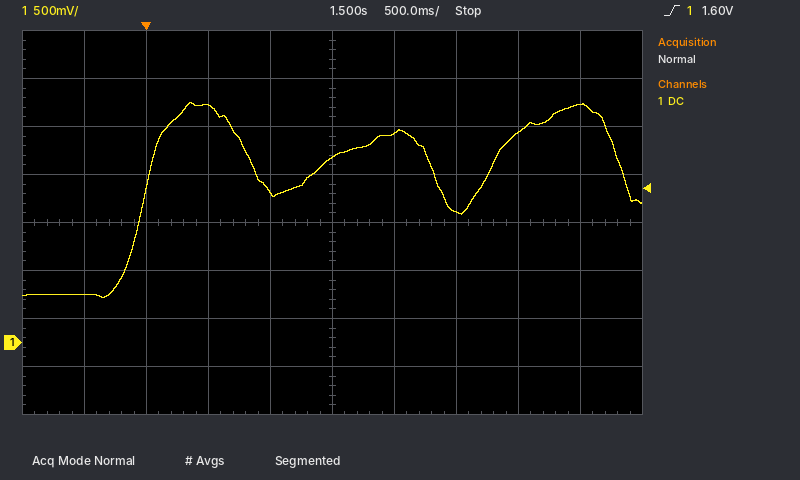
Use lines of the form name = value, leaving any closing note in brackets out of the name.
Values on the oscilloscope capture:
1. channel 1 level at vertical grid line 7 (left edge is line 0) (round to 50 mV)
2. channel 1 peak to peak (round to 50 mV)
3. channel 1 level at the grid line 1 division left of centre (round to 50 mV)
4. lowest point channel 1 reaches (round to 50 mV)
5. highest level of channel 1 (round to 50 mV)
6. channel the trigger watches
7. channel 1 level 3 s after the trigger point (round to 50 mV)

channel 1 level at vertical grid line 7 (left edge is line 0) = 1.35 V
channel 1 peak to peak = 2.05 V
channel 1 level at the grid line 1 division left of centre = 1.55 V
lowest point channel 1 reaches = 450 mV
highest level of channel 1 = 2.50 V
channel the trigger watches = channel 1
channel 1 level 3 s after the trigger point = 2.20 V
